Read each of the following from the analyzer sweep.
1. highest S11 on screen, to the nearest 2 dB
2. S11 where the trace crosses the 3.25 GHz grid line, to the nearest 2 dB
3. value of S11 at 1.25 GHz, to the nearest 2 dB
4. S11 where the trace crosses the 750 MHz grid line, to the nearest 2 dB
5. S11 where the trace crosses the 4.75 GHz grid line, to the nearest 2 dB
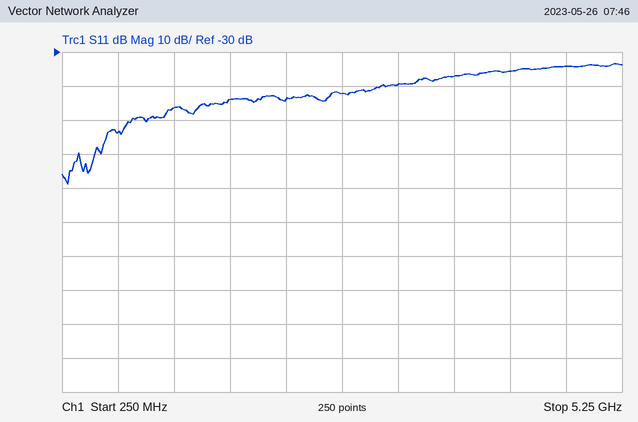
-34 dB
-40 dB
-46 dB
-54 dB
-34 dB
